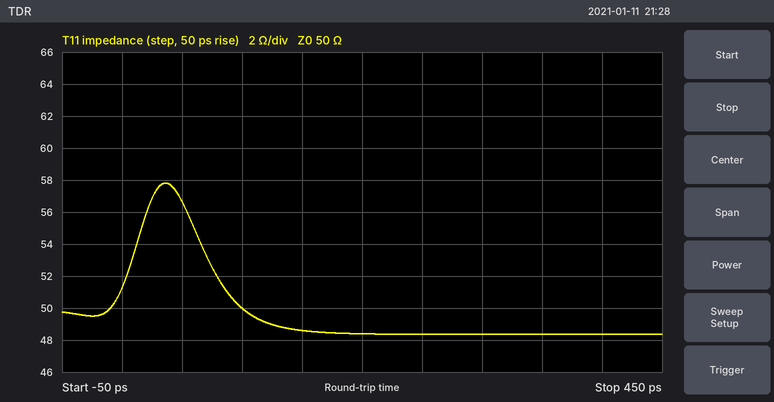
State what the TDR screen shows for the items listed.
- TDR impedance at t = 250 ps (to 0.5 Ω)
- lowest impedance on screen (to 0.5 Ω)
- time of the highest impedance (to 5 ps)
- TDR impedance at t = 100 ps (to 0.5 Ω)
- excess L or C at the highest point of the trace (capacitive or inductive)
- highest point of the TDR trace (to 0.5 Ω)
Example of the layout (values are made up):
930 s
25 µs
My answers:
48.5 Ω
48.5 Ω
35 ps
50.0 Ω
inductive
58.0 Ω
